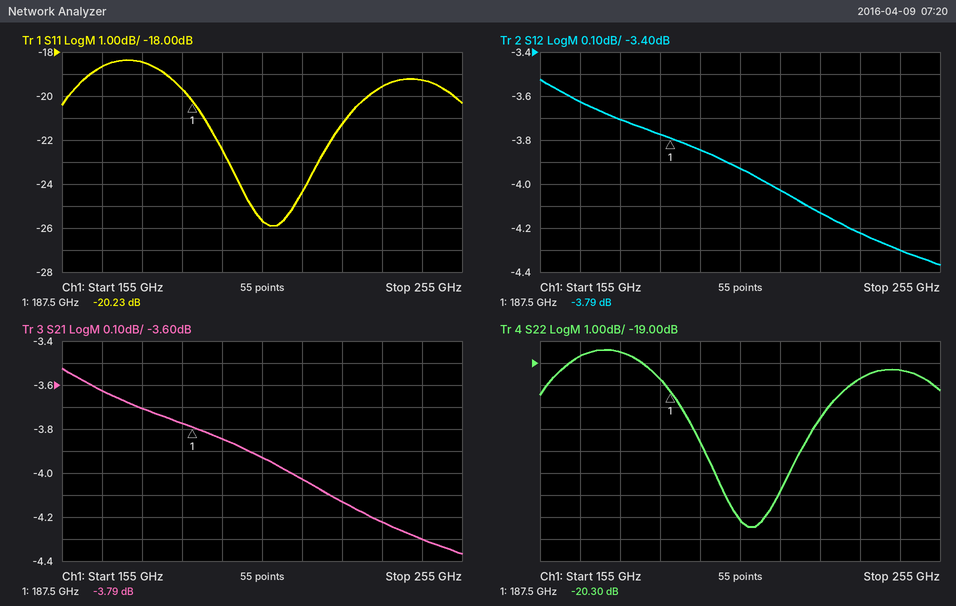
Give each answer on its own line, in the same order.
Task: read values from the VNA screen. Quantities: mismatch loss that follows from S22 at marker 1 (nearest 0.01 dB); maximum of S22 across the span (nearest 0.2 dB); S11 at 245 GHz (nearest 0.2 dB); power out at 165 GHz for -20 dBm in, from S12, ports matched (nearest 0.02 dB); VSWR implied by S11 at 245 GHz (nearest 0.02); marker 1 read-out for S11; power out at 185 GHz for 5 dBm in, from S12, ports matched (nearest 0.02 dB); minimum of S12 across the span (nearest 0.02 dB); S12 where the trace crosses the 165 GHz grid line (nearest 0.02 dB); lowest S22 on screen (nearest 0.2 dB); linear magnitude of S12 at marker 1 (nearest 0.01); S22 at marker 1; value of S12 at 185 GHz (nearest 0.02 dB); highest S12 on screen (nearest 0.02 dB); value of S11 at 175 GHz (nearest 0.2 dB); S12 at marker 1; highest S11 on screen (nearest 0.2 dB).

0.04 dB
-18.4 dB
-19.2 dB
-23.62 dBm
1.24
-20.23 dB
1.22 dBm
-4.36 dB
-3.62 dB
-26.4 dB
0.65
-20.30 dB
-3.78 dB
-3.52 dB
-18.4 dB
-3.79 dB
-18.4 dB
